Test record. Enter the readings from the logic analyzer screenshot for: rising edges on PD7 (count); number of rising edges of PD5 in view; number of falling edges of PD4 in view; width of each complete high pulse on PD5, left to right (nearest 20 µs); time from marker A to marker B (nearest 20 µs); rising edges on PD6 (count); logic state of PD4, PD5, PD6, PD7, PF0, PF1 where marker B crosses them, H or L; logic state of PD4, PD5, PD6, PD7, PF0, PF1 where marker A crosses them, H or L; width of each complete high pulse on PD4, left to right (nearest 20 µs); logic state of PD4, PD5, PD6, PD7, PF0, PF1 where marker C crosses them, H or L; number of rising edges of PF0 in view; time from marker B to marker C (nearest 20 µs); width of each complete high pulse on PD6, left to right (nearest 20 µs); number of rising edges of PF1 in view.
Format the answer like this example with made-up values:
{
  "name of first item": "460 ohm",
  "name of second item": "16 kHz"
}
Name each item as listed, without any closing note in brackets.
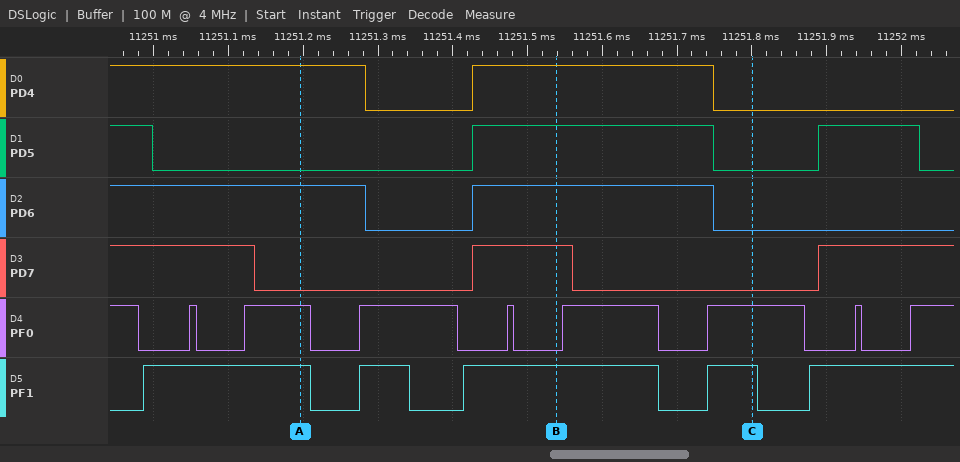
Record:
{
  "rising edges on PD7": "2",
  "number of rising edges of PD5 in view": "2",
  "number of falling edges of PD4 in view": "2",
  "width of each complete high pulse on PD5, left to right": "320 µs, 140 µs",
  "time from marker A to marker B": "340 µs",
  "rising edges on PD6": "1",
  "logic state of PD4, PD5, PD6, PD7, PF0, PF1 where marker B crosses them, H or L": "PD4=H, PD5=H, PD6=H, PD7=H, PF0=L, PF1=H",
  "logic state of PD4, PD5, PD6, PD7, PF0, PF1 where marker A crosses them, H or L": "PD4=H, PD5=L, PD6=H, PD7=L, PF0=H, PF1=H",
  "width of each complete high pulse on PD4, left to right": "320 µs",
  "logic state of PD4, PD5, PD6, PD7, PF0, PF1 where marker C crosses them, H or L": "PD4=L, PD5=L, PD6=L, PD7=L, PF0=H, PF1=H",
  "number of rising edges of PF0 in view": "8",
  "time from marker B to marker C": "260 µs",
  "width of each complete high pulse on PD6, left to right": "320 µs",
  "number of rising edges of PF1 in view": "5"
}
